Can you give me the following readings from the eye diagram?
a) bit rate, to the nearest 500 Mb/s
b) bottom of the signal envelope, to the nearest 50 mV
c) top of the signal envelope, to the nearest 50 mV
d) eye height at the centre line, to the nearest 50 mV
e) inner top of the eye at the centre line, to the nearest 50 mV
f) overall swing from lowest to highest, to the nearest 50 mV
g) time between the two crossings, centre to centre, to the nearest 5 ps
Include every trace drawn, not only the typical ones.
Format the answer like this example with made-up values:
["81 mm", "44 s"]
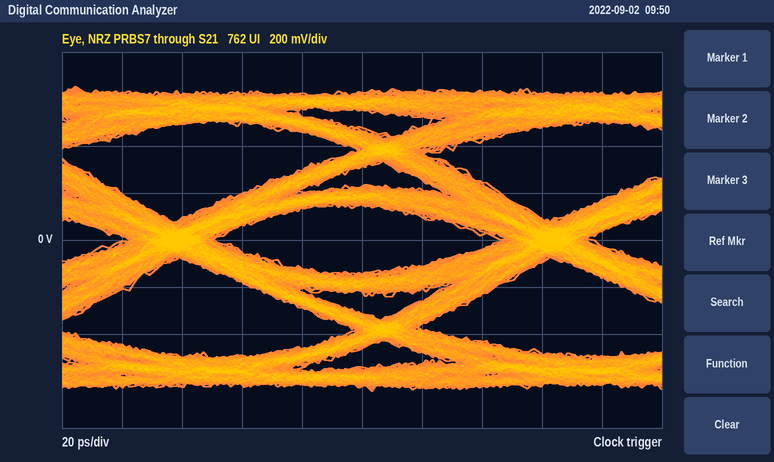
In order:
["8.0 Gb/s", "-650 mV", "650 mV", "300 mV", "150 mV", "1.30 V", "125 ps"]
